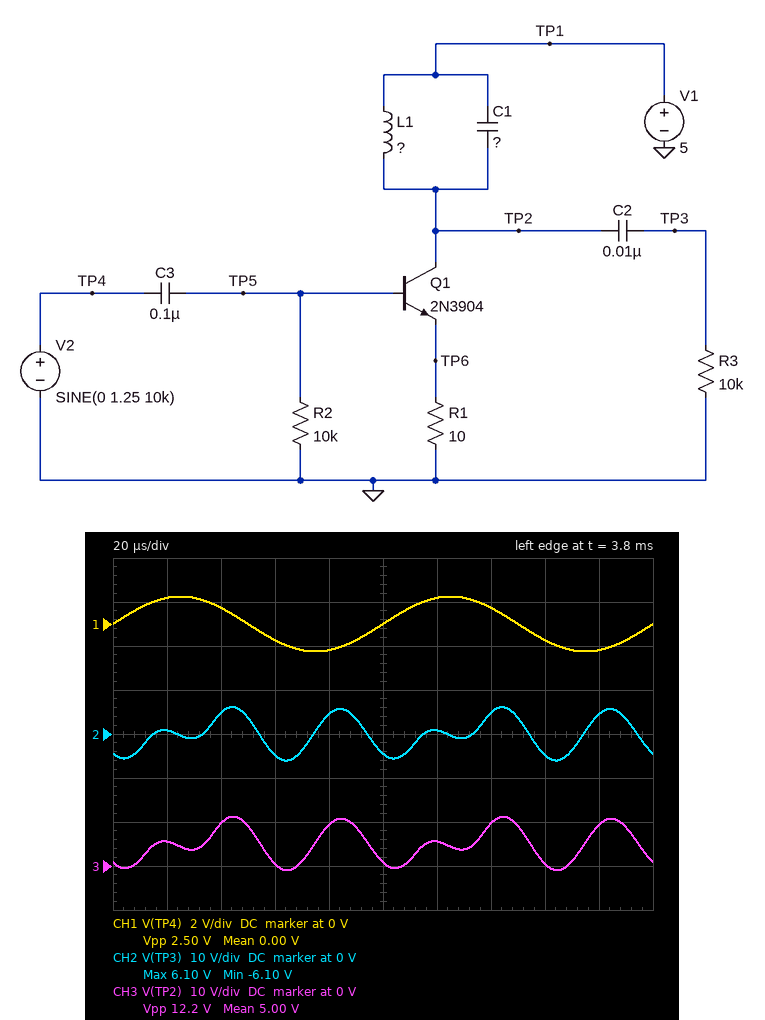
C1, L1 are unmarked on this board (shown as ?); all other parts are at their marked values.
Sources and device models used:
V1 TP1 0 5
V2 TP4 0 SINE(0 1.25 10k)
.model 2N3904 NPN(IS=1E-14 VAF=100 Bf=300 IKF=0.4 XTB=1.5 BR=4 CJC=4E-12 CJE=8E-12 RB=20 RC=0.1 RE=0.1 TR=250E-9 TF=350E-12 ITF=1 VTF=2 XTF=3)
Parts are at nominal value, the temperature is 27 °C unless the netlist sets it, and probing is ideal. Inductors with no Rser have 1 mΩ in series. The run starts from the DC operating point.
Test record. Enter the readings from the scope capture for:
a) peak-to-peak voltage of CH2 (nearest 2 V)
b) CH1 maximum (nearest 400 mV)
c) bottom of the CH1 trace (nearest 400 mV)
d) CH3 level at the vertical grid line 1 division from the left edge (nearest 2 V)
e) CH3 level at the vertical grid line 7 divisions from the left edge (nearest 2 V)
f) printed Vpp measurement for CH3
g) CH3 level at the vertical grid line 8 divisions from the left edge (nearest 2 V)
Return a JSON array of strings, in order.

["12 V", "1.2 V", "-1.2 V", "6 V", "10 V", "12.2 V", "0 V"]
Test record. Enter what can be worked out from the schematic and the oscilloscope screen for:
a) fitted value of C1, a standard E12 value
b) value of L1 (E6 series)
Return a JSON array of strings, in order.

["27 nF", "1.5 mH"]
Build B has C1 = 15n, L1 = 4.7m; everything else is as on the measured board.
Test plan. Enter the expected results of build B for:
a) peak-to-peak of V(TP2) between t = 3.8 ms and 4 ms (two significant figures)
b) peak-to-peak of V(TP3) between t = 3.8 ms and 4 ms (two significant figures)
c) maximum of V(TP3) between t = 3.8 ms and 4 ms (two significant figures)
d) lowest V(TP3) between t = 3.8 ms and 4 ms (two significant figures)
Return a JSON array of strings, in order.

["9.7 V", "9.8 V", "4.7 V", "-5.1 V"]
